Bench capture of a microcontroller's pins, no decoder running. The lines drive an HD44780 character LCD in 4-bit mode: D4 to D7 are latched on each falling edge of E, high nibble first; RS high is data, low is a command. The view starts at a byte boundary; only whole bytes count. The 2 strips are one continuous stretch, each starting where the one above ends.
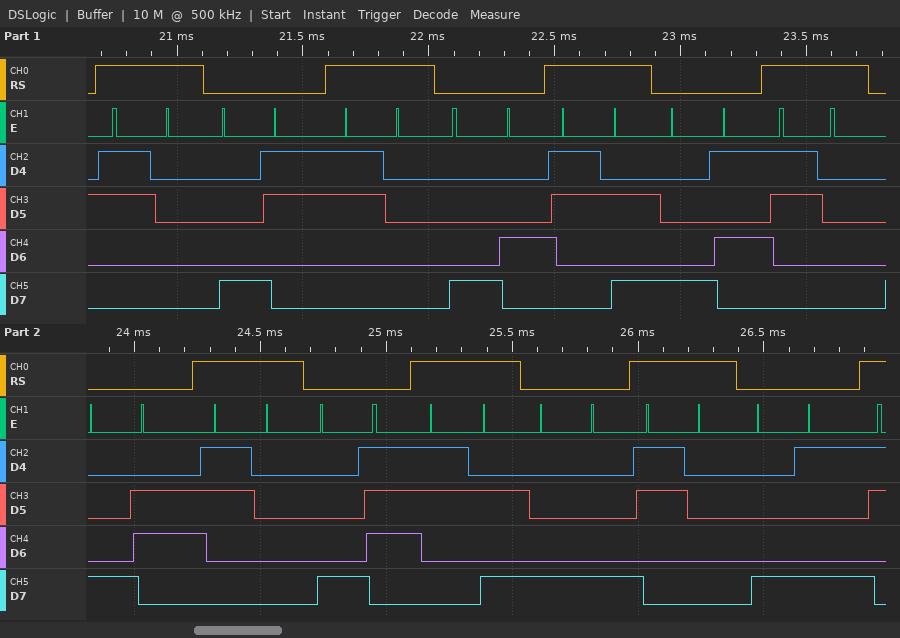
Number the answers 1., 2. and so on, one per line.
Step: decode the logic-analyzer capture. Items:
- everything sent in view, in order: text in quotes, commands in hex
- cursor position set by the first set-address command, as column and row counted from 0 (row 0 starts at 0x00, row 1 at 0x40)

1. "0" 0x83 "0" 0x84 ":" 0x85 "0" 0x86 "0" 0x87 ":" 0x88 "0" 0x89
2. column 3, row 0
